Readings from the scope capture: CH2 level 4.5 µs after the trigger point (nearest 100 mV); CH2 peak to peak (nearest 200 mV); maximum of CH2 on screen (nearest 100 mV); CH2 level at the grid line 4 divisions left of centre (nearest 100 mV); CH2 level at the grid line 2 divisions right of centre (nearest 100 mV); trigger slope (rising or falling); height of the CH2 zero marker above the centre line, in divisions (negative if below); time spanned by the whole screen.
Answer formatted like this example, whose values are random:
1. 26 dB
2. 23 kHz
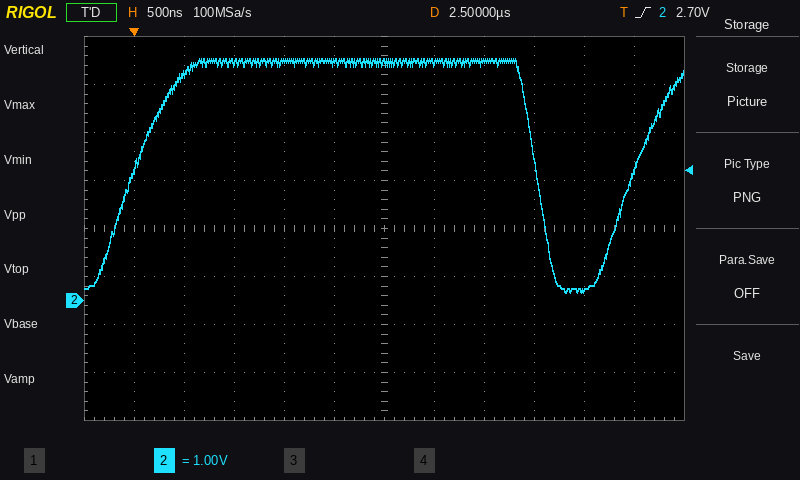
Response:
1. 200 mV
2. 4.8 V
3. 5.0 V
4. 4.7 V
5. 5.0 V
6. rising
7. -1.5 div
8. 6 µs
